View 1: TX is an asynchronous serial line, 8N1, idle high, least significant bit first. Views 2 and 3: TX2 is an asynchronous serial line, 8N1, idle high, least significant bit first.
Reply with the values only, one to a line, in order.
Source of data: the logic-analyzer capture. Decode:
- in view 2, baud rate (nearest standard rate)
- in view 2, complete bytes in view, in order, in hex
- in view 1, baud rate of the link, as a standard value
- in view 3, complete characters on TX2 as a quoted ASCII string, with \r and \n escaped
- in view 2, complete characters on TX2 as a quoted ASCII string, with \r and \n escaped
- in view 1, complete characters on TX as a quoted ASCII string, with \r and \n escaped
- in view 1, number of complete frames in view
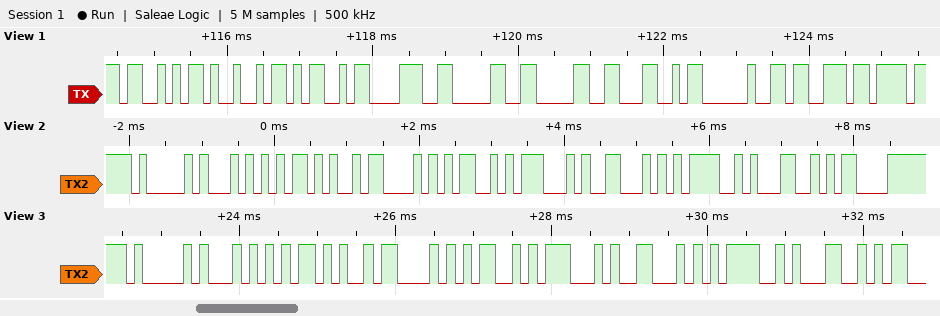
9600 baud
0x41 0x54 0x2B 0x43 0x4D 0x47 0x46 0x3D 0x31 0x0D
9600 baud
"AT+CMGF=1"
"AT+CMGF=1\r"
"SIM800L s"
9
